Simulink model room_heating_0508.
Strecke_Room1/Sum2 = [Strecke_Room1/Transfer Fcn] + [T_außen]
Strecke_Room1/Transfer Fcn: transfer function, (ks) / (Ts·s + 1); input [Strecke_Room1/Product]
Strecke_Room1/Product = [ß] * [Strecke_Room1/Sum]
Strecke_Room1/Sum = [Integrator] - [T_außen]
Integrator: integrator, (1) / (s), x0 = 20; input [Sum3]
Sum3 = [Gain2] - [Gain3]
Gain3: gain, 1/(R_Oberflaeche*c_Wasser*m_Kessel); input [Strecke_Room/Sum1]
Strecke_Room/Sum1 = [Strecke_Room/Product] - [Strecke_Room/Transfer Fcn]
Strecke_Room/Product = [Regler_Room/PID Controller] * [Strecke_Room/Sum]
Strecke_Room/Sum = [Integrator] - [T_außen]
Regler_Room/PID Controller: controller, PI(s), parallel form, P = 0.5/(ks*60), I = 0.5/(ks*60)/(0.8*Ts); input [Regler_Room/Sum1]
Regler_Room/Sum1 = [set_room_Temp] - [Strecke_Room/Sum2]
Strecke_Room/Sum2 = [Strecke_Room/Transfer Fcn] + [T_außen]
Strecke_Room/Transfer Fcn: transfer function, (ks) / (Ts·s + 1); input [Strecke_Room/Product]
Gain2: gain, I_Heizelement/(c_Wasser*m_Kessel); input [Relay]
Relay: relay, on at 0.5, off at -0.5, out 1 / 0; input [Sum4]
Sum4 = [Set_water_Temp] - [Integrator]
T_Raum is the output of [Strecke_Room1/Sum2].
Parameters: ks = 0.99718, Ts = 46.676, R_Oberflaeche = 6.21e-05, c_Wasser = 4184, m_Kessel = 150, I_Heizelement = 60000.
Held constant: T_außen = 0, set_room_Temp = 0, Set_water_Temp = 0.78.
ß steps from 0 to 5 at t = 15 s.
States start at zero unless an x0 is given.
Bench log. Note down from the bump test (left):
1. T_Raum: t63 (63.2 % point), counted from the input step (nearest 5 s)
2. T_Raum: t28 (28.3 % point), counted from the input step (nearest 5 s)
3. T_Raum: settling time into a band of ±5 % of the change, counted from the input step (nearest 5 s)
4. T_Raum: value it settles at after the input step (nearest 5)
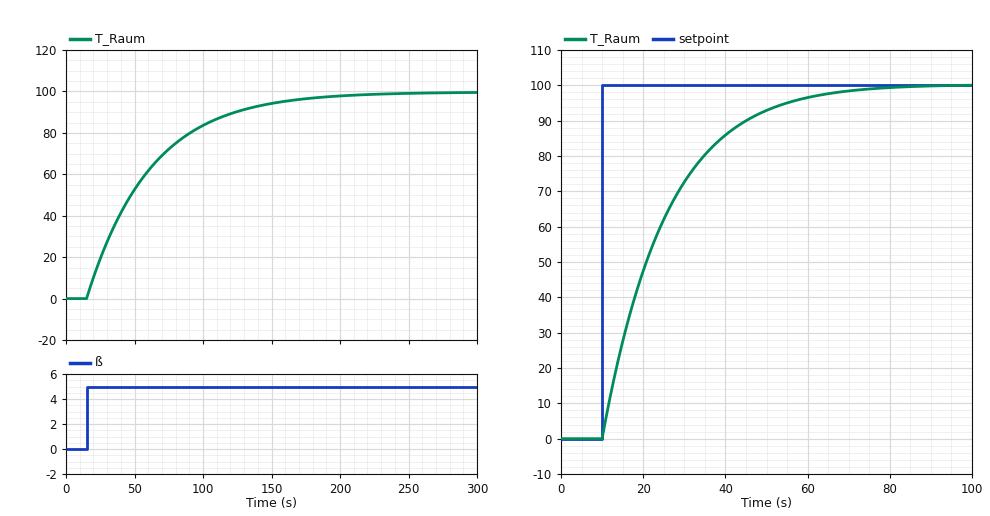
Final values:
45 s
15 s
140 s
100
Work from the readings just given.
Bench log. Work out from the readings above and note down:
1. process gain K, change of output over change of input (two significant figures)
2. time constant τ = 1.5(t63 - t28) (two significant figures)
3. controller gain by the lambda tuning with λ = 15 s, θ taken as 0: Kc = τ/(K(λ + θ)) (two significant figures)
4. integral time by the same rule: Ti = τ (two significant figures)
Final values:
20
45 s
0.15
45 s
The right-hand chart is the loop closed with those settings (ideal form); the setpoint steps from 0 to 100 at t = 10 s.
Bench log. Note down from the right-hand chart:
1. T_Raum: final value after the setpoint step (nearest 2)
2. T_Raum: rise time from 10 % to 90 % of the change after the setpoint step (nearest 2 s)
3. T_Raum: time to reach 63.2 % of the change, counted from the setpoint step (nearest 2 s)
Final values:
100
34 s
16 s
